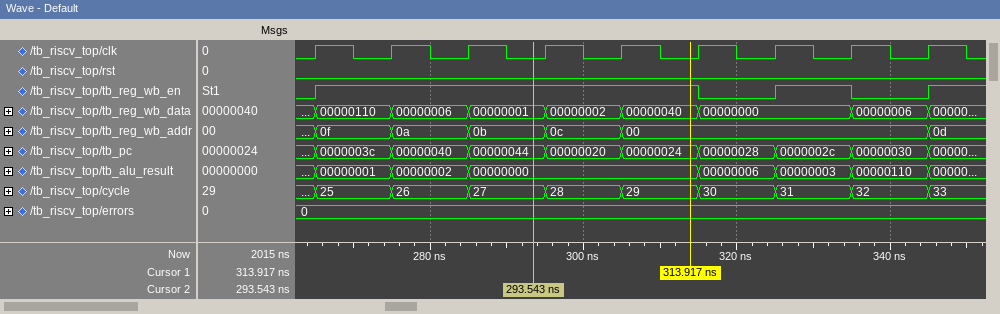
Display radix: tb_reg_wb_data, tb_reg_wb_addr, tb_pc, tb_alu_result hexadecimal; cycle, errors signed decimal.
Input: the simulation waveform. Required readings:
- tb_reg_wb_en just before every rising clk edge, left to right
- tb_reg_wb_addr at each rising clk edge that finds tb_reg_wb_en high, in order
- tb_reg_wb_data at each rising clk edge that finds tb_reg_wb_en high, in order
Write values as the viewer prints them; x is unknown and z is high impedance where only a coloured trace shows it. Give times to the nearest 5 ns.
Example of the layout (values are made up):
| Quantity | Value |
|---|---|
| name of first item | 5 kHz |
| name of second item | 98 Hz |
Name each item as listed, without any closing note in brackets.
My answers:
| Quantity | Value |
|---|---|
| tb_reg_wb_en just before every rising clk edge, left to right | 0 1 1 1 1 1 0 1 0 |
| tb_reg_wb_addr at each rising clk edge that finds tb_reg_wb_en high, in order | 0f, 0a, 0b, 0c, 00, 00 |
| tb_reg_wb_data at each rising clk edge that finds tb_reg_wb_en high, in order | 00000110, 00000006, 00000001, 00000002, 00000040, 00000000 |
